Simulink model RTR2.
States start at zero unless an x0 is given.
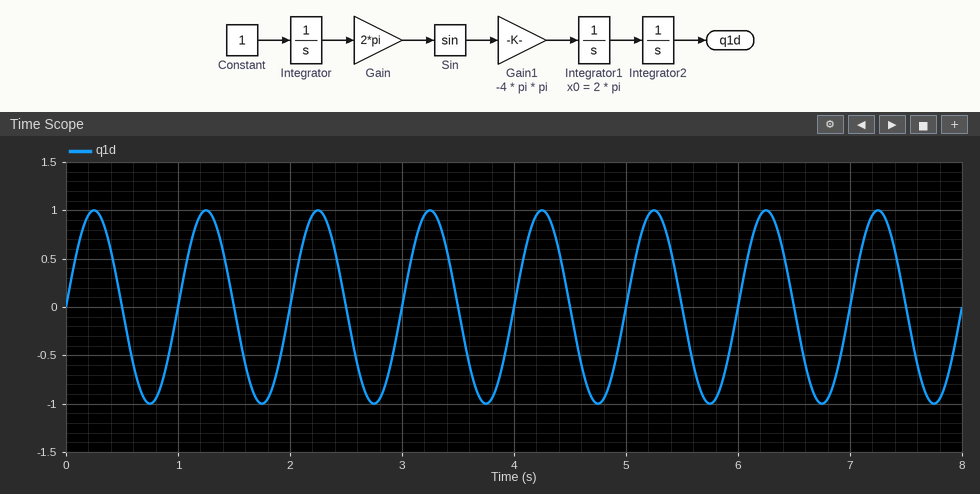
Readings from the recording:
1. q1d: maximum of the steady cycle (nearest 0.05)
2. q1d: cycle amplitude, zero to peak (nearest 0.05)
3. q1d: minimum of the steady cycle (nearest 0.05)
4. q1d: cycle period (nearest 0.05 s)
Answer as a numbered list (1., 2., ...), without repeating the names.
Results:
1. 1.00
2. 1.00
3. -1.00
4. 1.00 s
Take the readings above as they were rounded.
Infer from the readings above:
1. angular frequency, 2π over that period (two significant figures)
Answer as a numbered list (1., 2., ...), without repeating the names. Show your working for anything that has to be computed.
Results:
1. 2π / 1 = 6.3 rad/s
